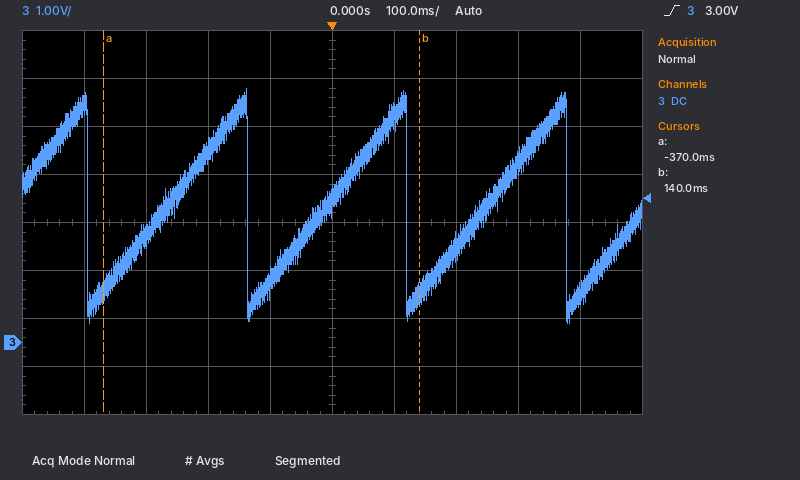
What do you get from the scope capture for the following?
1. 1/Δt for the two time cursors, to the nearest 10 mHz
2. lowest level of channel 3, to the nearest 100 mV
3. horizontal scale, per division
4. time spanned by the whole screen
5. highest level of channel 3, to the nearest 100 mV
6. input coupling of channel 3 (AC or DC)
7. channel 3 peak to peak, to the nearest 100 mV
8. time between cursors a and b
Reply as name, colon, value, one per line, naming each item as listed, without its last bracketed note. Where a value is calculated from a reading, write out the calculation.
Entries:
1/Δt for the two time cursors, to the nearest 10 mHz: 1 / 510 ms ≈ 1.96 Hz
lowest level of channel 3, to the nearest 100 mV: 400 mV
horizontal scale, per division: 100 ms
time spanned by the whole screen: 1 s
highest level of channel 3, to the nearest 100 mV: 5.3 V
input coupling of channel 3: DC
channel 3 peak to peak, to the nearest 100 mV: 5.3 V − (400 mV) = 4.9 V
time between cursors a and b: 140 ms − (-370 ms) = 510 ms
